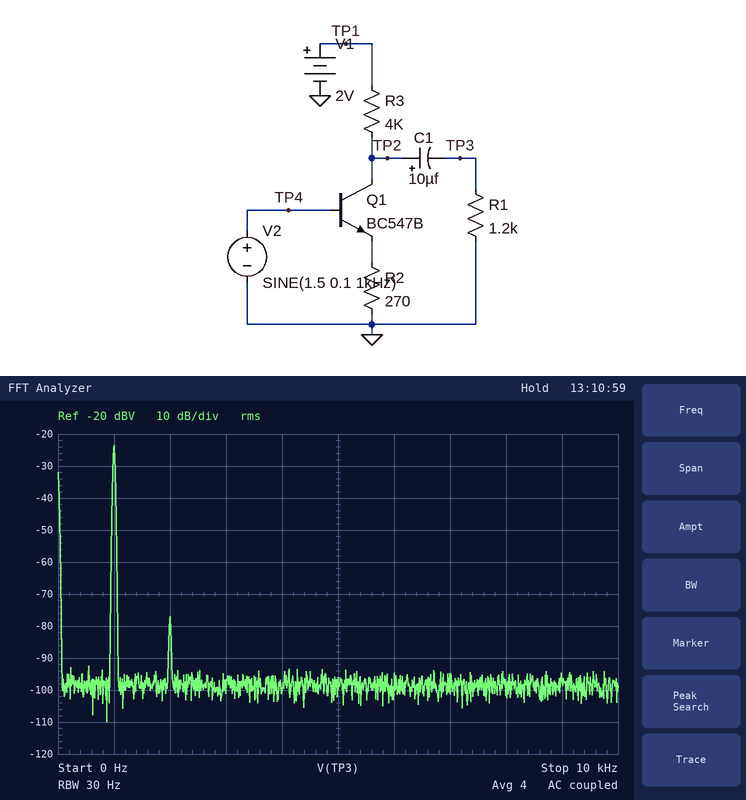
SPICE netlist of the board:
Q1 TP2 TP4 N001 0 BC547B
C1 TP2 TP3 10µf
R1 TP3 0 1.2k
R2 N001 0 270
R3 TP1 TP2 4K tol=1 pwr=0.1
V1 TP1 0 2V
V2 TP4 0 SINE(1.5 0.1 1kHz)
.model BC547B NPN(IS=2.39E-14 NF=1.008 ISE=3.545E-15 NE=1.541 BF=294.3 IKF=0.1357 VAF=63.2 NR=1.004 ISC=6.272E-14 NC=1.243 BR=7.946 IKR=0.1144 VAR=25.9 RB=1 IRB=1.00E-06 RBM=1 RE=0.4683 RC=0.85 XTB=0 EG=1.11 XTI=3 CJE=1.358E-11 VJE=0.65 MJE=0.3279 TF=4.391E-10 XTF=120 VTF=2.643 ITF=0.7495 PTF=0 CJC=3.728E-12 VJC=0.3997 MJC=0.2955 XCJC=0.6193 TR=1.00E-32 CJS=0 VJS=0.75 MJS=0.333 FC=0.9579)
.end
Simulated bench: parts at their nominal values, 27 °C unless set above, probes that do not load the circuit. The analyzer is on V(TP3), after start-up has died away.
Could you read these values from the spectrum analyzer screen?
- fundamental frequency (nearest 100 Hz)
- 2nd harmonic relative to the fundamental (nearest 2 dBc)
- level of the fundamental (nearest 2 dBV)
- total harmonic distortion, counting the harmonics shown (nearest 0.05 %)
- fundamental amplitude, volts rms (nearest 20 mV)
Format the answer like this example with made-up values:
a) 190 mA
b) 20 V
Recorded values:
a) 1.0 kHz
b) -54 dBc
c) -24 dBV
d) 0.20 %
e) 60 mV
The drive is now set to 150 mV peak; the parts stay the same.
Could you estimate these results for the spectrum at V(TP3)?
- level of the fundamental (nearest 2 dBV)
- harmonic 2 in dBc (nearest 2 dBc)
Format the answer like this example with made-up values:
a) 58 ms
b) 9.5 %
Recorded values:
a) -20 dBV
b) -50 dBc
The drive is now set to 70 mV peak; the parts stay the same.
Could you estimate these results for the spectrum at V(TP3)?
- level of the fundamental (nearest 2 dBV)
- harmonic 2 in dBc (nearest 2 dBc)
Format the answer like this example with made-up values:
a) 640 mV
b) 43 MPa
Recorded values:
a) -26 dBV
b) -56 dBc
